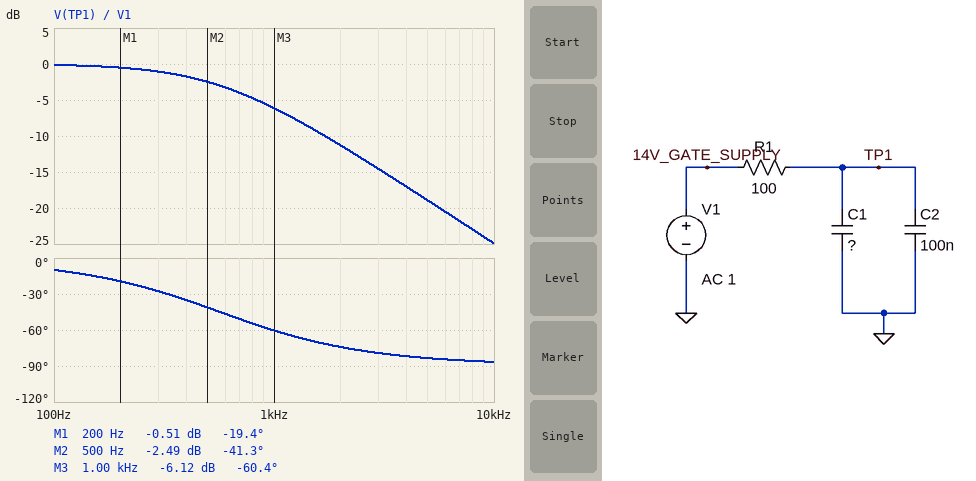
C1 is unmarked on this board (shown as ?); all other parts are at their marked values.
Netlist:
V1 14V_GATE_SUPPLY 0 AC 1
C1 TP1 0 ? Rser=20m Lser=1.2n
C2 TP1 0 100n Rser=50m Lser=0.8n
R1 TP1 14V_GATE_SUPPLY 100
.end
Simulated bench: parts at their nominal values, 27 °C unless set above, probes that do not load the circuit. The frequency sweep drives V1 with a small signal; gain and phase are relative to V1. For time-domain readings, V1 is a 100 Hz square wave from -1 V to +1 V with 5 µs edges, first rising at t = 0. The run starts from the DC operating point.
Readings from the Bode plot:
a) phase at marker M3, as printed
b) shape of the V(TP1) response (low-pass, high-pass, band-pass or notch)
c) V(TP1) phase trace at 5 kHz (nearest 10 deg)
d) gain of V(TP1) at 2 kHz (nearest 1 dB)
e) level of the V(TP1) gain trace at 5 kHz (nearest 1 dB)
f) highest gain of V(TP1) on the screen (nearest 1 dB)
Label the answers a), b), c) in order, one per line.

a) -60.4 deg
b) low-pass
c) -80 deg
d) -11 dB
e) -19 dB
f) 0 dB
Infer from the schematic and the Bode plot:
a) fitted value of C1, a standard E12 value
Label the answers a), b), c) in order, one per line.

a) 2.7 µF
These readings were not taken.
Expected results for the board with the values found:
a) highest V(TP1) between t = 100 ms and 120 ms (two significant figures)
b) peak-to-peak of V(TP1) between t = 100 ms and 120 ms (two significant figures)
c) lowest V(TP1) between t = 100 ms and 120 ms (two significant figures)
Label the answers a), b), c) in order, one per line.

a) 1.0 V
b) 2.0 V
c) -1.0 V
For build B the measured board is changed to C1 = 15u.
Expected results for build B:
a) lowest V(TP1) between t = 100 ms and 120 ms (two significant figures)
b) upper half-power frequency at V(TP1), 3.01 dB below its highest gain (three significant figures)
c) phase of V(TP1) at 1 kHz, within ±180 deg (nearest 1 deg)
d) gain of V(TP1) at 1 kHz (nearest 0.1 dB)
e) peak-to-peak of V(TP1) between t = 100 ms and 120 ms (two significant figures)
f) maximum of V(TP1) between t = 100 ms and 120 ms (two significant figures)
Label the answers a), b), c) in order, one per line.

a) -930 mV
b) 105 Hz
c) -84 deg
d) -19.6 dB
e) 1.9 V
f) 930 mV
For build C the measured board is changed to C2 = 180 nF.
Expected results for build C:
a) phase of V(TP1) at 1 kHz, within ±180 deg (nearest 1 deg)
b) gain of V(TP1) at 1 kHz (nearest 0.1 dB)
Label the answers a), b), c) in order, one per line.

a) -61 deg
b) -6.3 dB
